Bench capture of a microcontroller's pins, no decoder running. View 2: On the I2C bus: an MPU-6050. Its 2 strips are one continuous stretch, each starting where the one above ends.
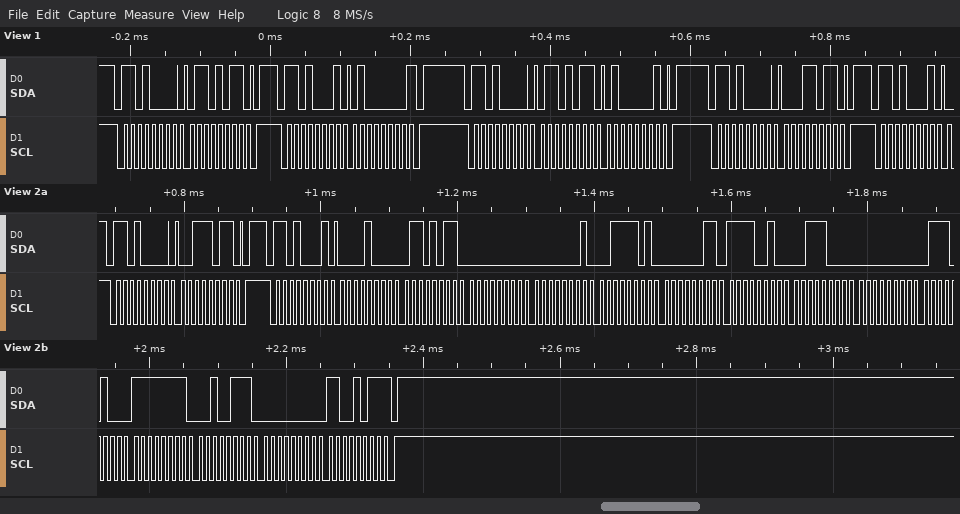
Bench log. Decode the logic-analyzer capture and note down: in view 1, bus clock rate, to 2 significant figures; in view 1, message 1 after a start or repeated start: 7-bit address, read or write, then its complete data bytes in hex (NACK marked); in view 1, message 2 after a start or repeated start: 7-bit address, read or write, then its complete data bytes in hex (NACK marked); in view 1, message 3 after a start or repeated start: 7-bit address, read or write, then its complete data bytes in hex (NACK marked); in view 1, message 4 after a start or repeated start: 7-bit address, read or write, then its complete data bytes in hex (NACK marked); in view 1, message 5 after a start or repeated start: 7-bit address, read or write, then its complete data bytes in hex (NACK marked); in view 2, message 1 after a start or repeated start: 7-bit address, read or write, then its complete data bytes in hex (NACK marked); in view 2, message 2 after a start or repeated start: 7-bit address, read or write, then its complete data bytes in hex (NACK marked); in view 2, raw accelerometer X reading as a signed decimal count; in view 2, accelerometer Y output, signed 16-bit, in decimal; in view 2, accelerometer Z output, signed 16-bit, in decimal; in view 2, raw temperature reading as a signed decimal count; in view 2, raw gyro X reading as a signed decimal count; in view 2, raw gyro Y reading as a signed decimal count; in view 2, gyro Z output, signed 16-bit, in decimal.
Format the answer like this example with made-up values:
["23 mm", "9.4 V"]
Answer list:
["100 kHz", "0x68 write: 6B", "0x68 read: 40 NACK", "0x68 write: 6B 41", "0x68 write: 1B", "0x68 read", "0x68 write: 3B", "0x68 read: 08 6B 00 01 3D 03 F2 38 00 74 FF 27 00 CB NACK", "2155", "1", "15619", "-3528", "116", "-217", "203"]
